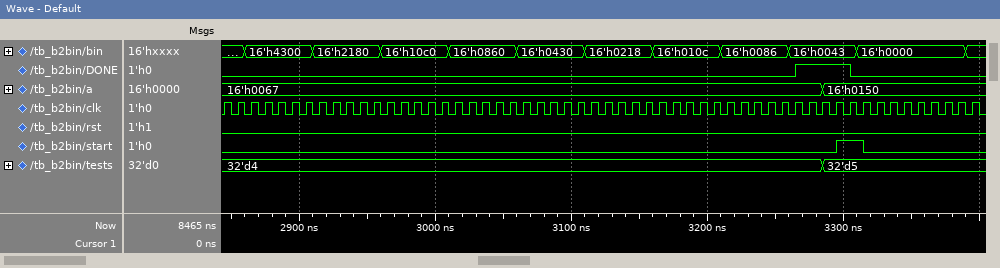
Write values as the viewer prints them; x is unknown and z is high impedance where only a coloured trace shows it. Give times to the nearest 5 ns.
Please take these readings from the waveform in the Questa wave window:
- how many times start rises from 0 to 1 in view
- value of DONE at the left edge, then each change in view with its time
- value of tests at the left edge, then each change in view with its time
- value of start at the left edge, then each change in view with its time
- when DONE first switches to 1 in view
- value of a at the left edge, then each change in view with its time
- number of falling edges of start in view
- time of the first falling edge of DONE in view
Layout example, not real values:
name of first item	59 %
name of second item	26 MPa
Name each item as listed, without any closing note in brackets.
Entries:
how many times start rises from 0 to 1 in view	1
value of DONE at the left edge, then each change in view with its time	0, 1 at 3265 ns, 0 at 3305 ns
value of tests at the left edge, then each change in view with its time	32'd4, 32'd5 at 3285 ns
value of start at the left edge, then each change in view with its time	0, 1 at 3295 ns, 0 at 3315 ns
when DONE first switches to 1 in view	3265 ns
value of a at the left edge, then each change in view with its time	16'h0067, 16'h0150 at 3285 ns
number of falling edges of start in view	1
time of the first falling edge of DONE in view	3305 ns
